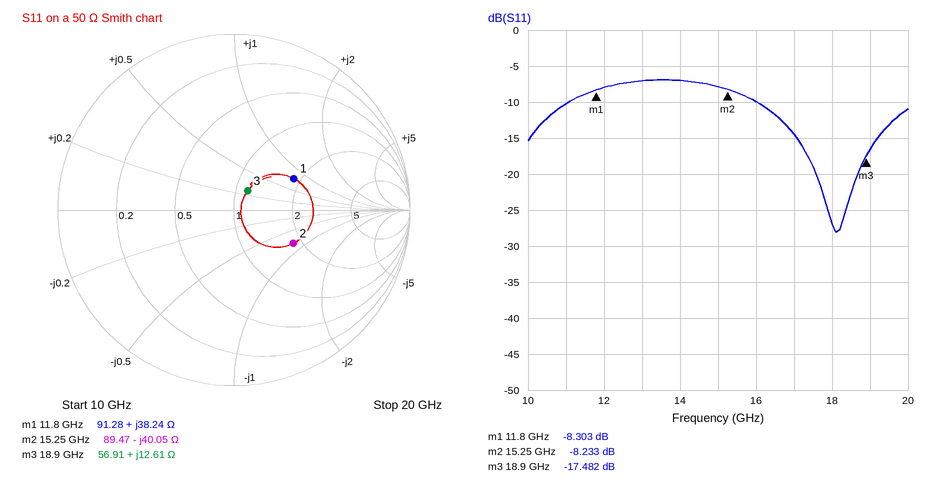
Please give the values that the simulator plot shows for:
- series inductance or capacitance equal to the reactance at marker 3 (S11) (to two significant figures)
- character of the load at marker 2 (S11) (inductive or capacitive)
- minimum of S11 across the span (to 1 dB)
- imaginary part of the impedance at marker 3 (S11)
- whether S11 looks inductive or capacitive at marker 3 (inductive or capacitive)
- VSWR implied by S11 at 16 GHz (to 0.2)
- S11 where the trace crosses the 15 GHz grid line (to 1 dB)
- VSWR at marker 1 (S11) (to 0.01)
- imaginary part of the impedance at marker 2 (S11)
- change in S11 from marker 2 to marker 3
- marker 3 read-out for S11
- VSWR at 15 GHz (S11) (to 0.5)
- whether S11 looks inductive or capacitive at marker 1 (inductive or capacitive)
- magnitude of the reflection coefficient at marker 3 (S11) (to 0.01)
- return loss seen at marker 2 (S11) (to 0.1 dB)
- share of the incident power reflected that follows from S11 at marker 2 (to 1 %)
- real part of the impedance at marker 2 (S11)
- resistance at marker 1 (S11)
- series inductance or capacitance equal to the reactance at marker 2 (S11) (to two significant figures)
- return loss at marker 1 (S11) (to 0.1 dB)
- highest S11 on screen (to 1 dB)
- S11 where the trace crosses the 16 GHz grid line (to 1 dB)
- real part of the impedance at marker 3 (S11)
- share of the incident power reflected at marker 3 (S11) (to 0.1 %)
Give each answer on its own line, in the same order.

110 pH
capacitive
-28 dB
+12.61 Ω
inductive
2.0
-8 dB
2.25
-40.05 Ω
-9.249 dB
-17.482 dB
2.5
inductive
0.13
8.2 dB
15 %
89.47 Ω
91.28 Ω
260 fF
8.3 dB
-7 dB
-10 dB
56.91 Ω
1.8 %
